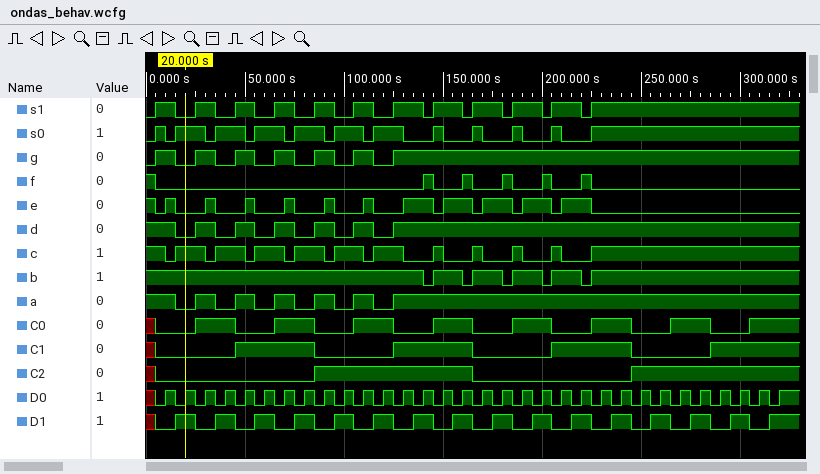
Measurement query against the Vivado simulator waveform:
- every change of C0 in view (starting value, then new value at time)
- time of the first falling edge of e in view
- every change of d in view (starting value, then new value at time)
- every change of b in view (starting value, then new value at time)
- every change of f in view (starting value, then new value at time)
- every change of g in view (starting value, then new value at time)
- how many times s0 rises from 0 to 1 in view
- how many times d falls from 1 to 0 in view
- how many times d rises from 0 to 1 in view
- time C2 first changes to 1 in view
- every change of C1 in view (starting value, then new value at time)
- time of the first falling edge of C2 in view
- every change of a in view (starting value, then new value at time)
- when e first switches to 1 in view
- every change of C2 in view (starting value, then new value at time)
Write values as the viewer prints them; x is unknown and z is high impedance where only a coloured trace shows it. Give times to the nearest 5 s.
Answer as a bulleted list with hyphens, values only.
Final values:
- x, 0 at 5 s, 1 at 25 s, 0 at 45 s, 1 at 65 s, 0 at 85 s, 1 at 105 s, 0 at 125 s, 1 at 145 s, 0 at 165 s, 1 at 185 s, 0 at 205 s, 1 at 225 s, 0 at 245 s, 1 at 265 s, 0 at 285 s, 1 at 305 s
- 5 s
- 1, 0 at 15 s, 1 at 25 s, 0 at 35 s, 1 at 45 s, 0 at 55 s, 1 at 65 s, 0 at 75 s, 1 at 85 s, 0 at 95 s, 1 at 105 s, 0 at 115 s, 1 at 125 s
- 1, 0 at 140 s, 1 at 145 s, 0 at 160 s, 1 at 165 s, 0 at 180 s, 1 at 185 s, 0 at 200 s, 1 at 205 s, 0 at 220 s, 1 at 225 s
- 1, 0 at 5 s, 1 at 140 s, 0 at 145 s, 1 at 160 s, 0 at 165 s, 1 at 180 s, 0 at 185 s, 1 at 200 s, 0 at 205 s, 1 at 220 s, 0 at 225 s
- 0, 1 at 5 s, 0 at 15 s, 1 at 25 s, 0 at 35 s, 1 at 45 s, 0 at 55 s, 1 at 65 s, 0 at 75 s, 1 at 85 s, 0 at 95 s, 1 at 105 s, 0 at 115 s, 1 at 125 s
- 12
- 6
- 6
- 85 s
- x, 0 at 5 s, 1 at 45 s, 0 at 85 s, 1 at 125 s, 0 at 165 s, 1 at 205 s, 0 at 245 s, 1 at 285 s
- 165 s
- 1, 0 at 15 s, 1 at 25 s, 0 at 35 s, 1 at 45 s, 0 at 55 s, 1 at 65 s, 0 at 75 s, 1 at 85 s, 0 at 95 s, 1 at 105 s, 0 at 115 s, 1 at 125 s
- 10 s
- x, 0 at 5 s, 1 at 85 s, 0 at 165 s, 1 at 245 s
